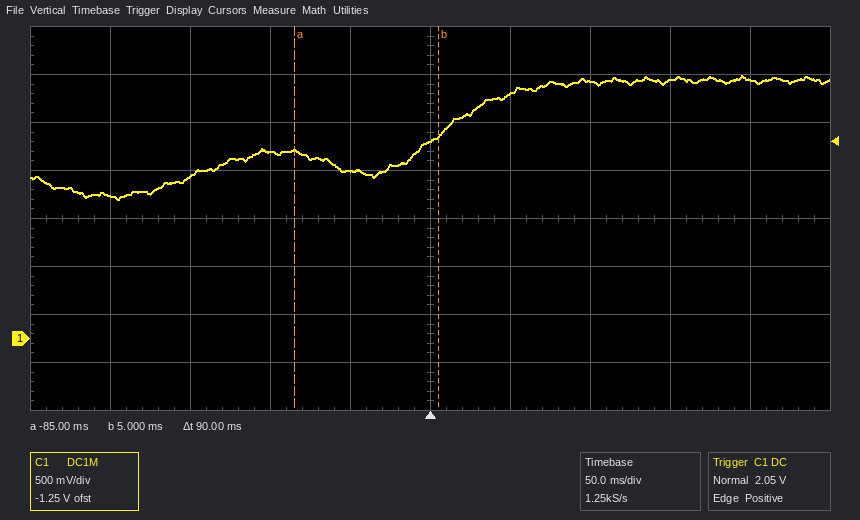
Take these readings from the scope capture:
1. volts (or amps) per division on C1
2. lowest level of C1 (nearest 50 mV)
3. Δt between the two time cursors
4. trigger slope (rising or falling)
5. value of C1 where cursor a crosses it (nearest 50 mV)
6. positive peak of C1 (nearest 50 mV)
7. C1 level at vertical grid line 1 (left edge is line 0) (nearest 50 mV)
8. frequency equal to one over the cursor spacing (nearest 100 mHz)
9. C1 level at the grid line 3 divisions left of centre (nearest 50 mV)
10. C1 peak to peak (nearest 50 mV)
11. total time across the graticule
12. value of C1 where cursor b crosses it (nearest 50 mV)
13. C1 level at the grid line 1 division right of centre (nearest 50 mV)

500 mV
1.45 V
90 ms
rising
1.95 V
2.75 V
1.50 V
11.1 Hz
1.70 V
1.30 V
500 ms
2.10 V
2.55 V
